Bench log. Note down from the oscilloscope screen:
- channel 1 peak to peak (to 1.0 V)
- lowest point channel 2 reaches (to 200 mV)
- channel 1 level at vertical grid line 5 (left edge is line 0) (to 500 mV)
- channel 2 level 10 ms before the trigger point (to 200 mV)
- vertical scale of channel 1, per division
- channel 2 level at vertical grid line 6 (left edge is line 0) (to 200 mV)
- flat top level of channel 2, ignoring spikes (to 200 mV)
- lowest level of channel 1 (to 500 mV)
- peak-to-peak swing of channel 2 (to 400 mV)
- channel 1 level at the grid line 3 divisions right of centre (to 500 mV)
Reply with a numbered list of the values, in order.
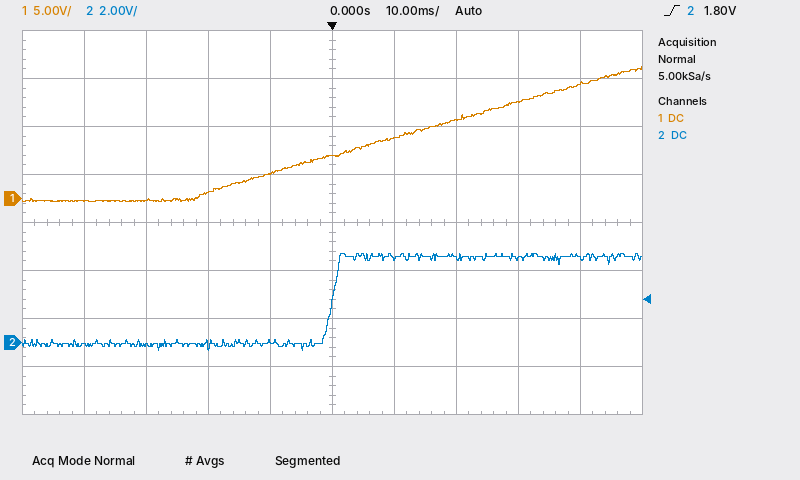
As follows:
1. 14.0 V
2. -400 mV
3. 4.5 V
4. 0.0 V
5. 5 V
6. 3.6 V
7. 3.6 V
8. -500 mV
9. 4.0 V
10. 10.0 V
